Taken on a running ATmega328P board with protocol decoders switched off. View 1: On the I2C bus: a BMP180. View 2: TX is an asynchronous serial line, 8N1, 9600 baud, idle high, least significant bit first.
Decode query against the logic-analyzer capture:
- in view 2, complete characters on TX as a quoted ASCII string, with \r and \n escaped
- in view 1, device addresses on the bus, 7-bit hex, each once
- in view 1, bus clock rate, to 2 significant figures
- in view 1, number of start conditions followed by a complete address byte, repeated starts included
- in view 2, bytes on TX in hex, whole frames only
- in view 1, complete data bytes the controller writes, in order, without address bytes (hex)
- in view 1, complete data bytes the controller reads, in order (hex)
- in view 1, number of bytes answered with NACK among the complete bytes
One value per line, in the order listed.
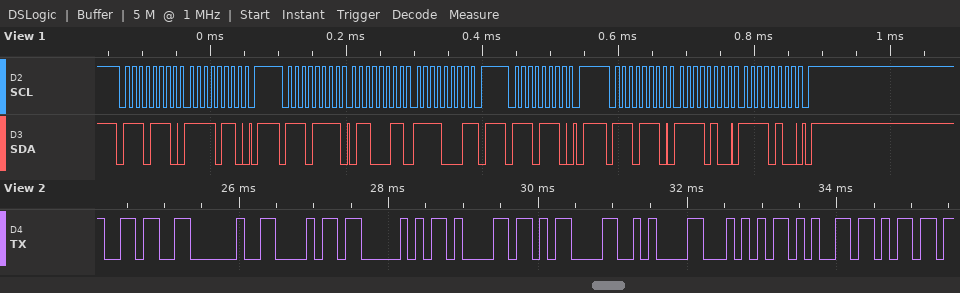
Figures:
"6 hPa\r\nTem"
0x77
100 kHz
4
36 20 68 50 61 0D 0A 54 65 6D
F6 F4 F4
63 F1
1
